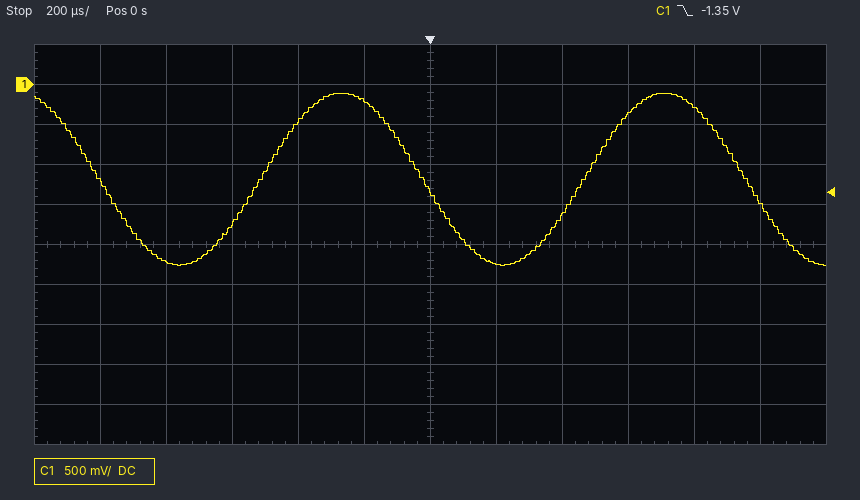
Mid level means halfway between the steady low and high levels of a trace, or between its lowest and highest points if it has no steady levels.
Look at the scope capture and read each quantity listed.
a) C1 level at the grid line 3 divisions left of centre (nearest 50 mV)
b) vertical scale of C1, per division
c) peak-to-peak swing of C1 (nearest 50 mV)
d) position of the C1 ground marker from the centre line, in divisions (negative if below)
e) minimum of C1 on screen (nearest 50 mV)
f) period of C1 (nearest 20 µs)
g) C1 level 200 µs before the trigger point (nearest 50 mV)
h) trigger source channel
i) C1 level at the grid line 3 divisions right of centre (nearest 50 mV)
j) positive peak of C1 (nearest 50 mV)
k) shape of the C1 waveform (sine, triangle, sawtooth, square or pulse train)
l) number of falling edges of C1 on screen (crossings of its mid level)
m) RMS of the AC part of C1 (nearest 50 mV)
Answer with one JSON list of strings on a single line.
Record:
["-1.75 V", "500 mV", "2.15 V", "+4.0 div", "-2.25 V", "980 µs", "-200 mV", "C1", "-400 mV", "-100 mV", "sine", "3", "750 mV"]
